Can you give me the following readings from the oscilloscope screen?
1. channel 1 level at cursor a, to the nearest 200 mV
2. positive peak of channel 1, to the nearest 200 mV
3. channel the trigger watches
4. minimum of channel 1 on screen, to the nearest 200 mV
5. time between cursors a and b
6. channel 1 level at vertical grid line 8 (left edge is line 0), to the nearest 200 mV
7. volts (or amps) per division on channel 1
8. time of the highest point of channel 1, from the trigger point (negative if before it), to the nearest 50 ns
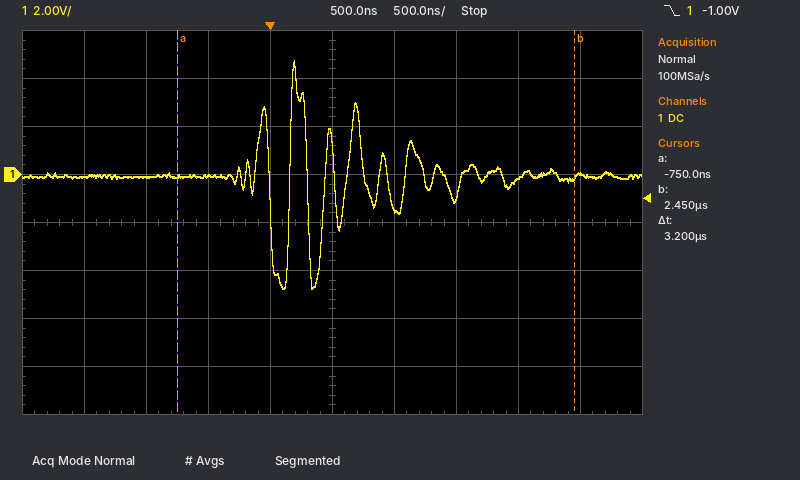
0.0 V
4.8 V
channel 1
-4.8 V
3.2 µs
-200 mV
2 V
+200 ns
